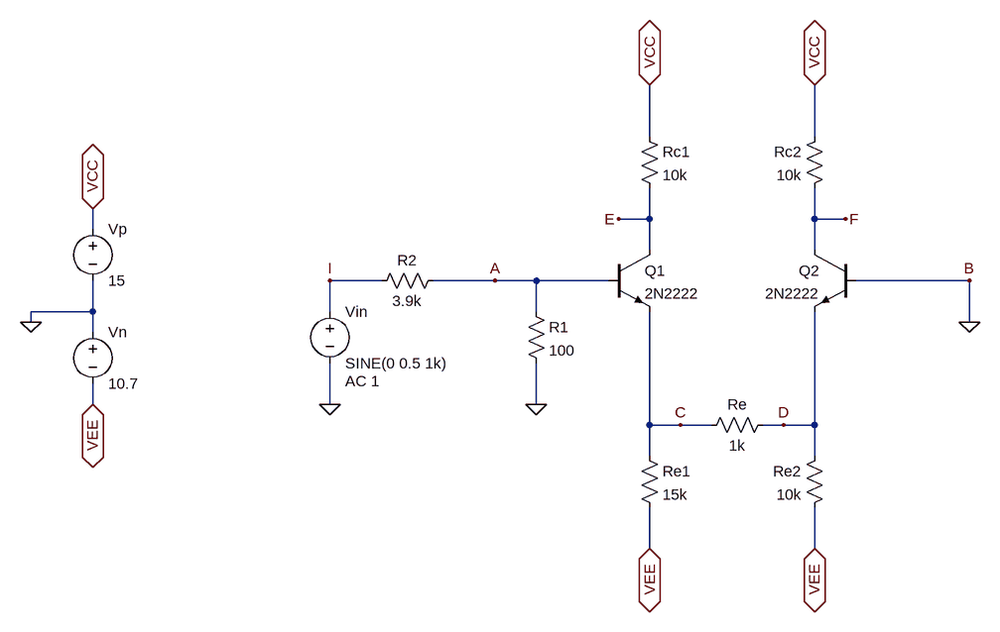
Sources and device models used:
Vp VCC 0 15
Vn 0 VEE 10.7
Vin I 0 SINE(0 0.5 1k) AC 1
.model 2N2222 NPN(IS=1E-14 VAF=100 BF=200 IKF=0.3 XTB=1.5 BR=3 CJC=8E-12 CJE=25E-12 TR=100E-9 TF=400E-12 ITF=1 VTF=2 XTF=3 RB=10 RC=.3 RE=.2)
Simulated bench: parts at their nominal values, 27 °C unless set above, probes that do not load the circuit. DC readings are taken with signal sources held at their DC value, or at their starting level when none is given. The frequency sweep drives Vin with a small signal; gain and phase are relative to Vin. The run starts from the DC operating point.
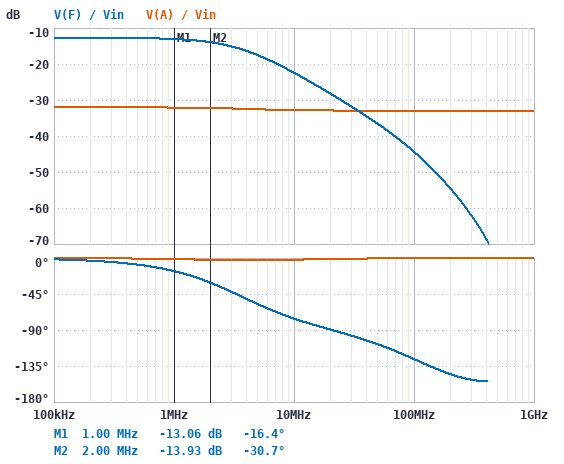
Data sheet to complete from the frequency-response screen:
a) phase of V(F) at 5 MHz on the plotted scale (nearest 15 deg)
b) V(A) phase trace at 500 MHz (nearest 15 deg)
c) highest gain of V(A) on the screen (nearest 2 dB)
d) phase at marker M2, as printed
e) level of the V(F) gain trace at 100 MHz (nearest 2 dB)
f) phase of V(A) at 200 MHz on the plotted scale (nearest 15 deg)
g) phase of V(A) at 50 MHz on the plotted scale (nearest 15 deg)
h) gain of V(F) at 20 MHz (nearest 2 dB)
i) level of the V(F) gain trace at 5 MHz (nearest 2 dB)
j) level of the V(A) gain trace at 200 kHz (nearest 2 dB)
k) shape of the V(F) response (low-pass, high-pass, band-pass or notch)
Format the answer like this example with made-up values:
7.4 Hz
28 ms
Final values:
-60 deg
0 deg
-32 dB
-30.7 deg
-44 dB
0 deg
0 deg
-28 dB
-18 dB
-32 dB
low-pass
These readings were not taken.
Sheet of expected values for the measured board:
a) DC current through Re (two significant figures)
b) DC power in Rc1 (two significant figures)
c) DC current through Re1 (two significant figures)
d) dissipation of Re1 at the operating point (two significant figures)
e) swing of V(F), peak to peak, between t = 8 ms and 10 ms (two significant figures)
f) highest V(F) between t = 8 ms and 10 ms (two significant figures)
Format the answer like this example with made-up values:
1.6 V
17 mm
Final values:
10 µA
4.6 mW
670 µA
6.7 mW
230 mV
5.2 V
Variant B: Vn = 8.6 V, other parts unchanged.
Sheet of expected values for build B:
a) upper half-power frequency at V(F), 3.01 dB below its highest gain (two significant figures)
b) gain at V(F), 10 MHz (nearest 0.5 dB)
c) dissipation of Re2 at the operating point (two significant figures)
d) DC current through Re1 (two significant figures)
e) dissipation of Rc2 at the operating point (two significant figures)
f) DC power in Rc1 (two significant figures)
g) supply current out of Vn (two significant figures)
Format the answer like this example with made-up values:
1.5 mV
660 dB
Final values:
3.9 MHz
-22.0 dB
6.3 mW
530 µA
6.1 mW
2.9 mW
1.3 mA
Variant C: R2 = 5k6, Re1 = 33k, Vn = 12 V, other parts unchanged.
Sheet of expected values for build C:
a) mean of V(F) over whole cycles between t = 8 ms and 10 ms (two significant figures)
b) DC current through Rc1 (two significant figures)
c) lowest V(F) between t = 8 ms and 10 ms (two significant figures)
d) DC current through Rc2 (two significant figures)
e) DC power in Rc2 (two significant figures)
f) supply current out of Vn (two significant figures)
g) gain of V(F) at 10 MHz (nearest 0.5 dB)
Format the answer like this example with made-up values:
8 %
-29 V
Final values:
4.0 V
370 µA
3.9 V
1.1 mA
12 mW
1.5 mA
-26.0 dB
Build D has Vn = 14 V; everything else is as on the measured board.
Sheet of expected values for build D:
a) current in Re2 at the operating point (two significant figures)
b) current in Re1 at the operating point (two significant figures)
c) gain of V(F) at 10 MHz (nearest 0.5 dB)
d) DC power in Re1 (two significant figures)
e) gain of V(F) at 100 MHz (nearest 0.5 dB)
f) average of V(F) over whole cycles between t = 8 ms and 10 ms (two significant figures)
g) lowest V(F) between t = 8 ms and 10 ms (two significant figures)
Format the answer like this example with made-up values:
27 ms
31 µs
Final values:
1.3 mA
890 µA
-24.5 dB
12 mW
-46.0 dB
1.8 V
1.7 V
